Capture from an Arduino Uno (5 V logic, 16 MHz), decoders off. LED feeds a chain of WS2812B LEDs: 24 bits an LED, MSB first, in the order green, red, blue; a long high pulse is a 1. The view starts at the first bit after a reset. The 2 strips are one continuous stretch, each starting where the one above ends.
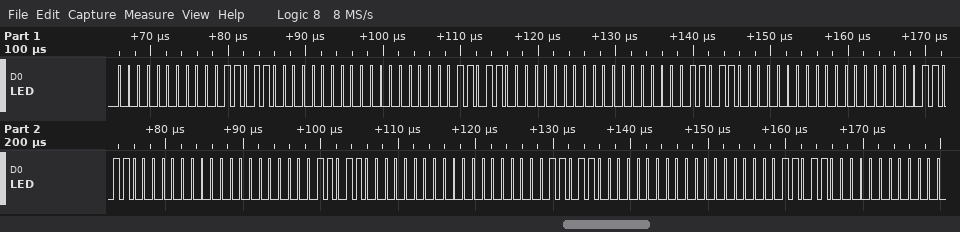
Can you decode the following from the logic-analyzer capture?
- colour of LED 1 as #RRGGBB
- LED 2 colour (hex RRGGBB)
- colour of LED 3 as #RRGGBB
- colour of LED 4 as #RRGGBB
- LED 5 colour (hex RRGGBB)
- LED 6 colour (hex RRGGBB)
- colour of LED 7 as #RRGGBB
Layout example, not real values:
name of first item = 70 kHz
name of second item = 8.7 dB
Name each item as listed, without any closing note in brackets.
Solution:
colour of LED 1 as #RRGGBB = #1B0000
LED 2 colour = #1B0000
colour of LED 3 as #RRGGBB = #1B0000
colour of LED 4 as #RRGGBB = #1B0000
LED 5 colour = #1B0000
LED 6 colour = #1B0000
colour of LED 7 as #RRGGBB = #1B0000
